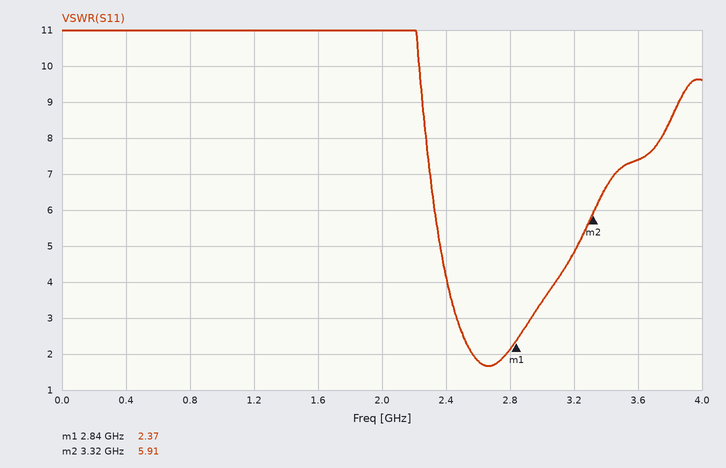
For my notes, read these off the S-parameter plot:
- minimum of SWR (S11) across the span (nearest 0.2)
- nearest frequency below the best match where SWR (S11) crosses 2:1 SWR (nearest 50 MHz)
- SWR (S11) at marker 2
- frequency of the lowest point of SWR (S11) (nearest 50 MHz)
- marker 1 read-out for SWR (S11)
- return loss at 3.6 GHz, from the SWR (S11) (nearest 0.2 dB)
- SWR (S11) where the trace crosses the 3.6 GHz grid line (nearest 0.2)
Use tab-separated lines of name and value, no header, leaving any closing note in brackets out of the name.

minimum of SWR (S11) across the span	1.6
nearest frequency below the best match where SWR (S11) crosses 2:1 SWR	2.55 GHz
SWR (S11) at marker 2	5.91
frequency of the lowest point of SWR (S11)	2.65 GHz
marker 1 read-out for SWR	2.37
return loss at 3.6 GHz, from the SWR (S11)	2.4 dB
SWR (S11) where the trace crosses the 3.6 GHz grid line	7.4
